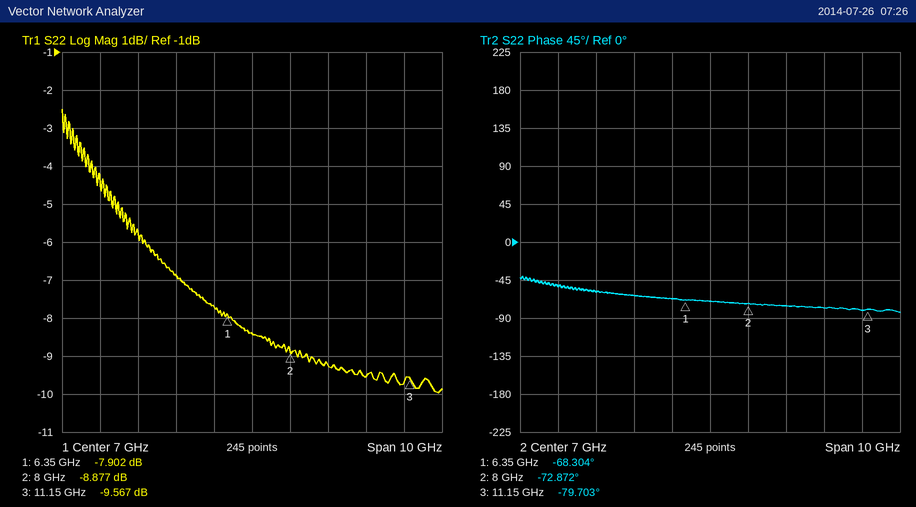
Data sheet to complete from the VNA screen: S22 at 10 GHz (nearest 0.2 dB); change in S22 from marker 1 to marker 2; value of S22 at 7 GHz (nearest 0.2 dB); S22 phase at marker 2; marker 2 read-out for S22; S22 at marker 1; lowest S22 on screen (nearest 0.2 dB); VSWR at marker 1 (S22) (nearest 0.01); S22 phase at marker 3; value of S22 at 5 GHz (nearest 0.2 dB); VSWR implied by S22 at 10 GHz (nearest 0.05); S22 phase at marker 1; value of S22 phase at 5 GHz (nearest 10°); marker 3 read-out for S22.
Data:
-9.6 dB
-0.975 dB
-8.4 dB
-72.872°
-8.877 dB
-7.902 dB
-10.0 dB
2.35
-79.703°
-6.8 dB
2.00
-68.304°
-60°
-9.567 dB
